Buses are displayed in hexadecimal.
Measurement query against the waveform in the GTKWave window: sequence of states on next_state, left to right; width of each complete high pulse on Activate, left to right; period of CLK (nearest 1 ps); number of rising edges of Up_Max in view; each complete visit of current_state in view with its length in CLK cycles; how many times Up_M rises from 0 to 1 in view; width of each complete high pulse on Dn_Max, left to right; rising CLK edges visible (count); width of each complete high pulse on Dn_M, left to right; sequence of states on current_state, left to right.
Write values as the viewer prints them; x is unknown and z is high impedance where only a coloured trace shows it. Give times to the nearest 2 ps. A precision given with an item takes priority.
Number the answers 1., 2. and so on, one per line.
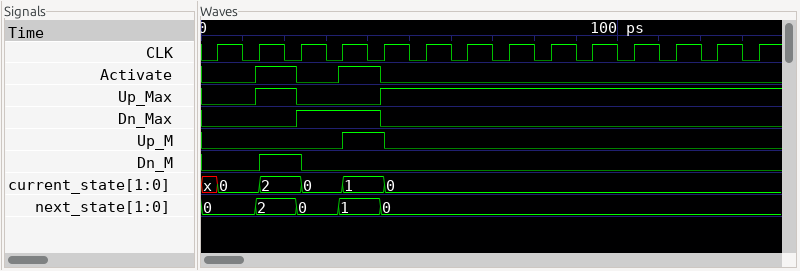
1. 0, 2, 0, 1, 0
2. 10 ps, 10 ps
3. 10 ps
4. 2
5. 0: 1, 2: 1, 0: 1, 1: 1
6. 1
7. 20 ps
8. 14
9. 10 ps
10. x, 0, 2, 0, 1, 0
